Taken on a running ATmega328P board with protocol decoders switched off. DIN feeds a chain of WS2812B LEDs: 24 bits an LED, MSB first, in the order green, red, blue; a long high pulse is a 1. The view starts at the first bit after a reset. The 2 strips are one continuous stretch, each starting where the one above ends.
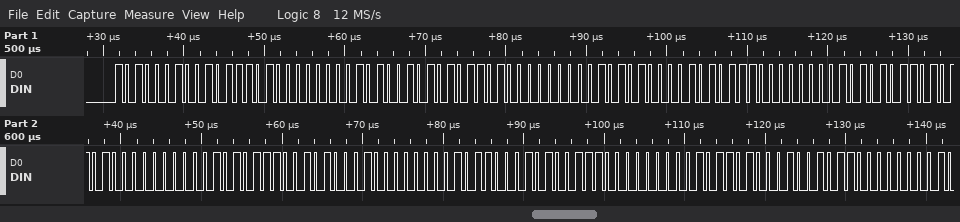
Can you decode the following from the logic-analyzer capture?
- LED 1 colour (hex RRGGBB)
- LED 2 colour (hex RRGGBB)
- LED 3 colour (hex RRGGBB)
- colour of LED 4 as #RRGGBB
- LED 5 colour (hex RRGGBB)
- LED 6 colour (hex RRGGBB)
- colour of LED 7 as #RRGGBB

#5DA200
#5AA500
#57A800
#54AB00
#51AE00
#4EB100
#4BB400
